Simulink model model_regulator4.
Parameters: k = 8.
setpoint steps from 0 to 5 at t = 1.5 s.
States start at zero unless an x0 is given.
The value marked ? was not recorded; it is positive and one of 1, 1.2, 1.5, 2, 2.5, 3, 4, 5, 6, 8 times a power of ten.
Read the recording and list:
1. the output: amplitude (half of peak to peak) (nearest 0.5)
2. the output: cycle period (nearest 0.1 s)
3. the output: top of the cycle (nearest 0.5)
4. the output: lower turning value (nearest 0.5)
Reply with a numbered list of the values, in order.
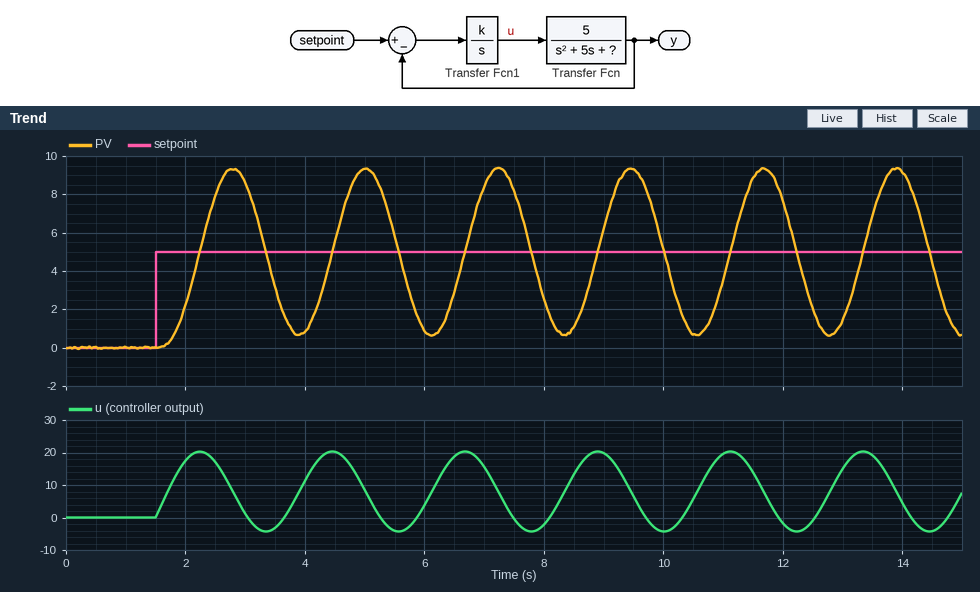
1. 4.5
2. 2.2 s
3. 9.5
4. 0.5
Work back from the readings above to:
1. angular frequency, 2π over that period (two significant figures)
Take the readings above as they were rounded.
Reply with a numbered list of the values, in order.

1. 2.9 rad/s
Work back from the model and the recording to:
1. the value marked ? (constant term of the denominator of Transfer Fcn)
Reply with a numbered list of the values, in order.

1. 8
